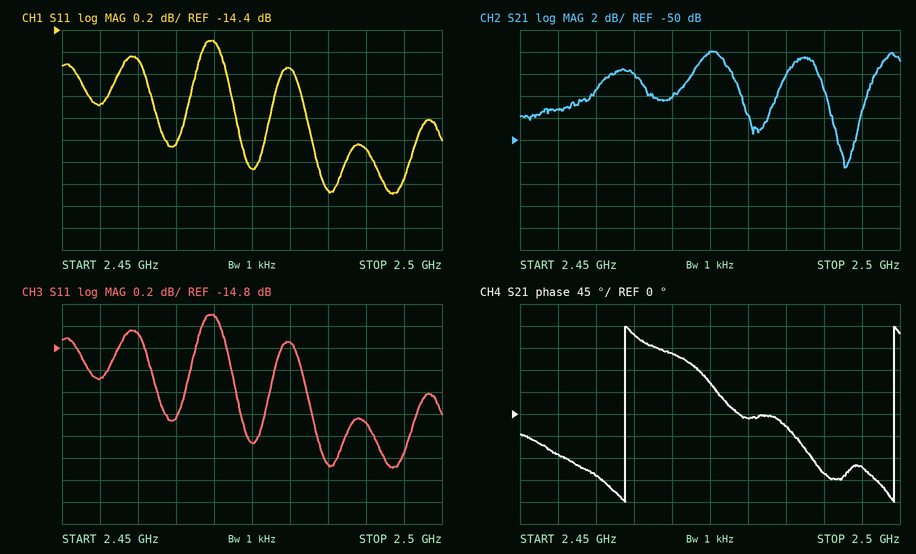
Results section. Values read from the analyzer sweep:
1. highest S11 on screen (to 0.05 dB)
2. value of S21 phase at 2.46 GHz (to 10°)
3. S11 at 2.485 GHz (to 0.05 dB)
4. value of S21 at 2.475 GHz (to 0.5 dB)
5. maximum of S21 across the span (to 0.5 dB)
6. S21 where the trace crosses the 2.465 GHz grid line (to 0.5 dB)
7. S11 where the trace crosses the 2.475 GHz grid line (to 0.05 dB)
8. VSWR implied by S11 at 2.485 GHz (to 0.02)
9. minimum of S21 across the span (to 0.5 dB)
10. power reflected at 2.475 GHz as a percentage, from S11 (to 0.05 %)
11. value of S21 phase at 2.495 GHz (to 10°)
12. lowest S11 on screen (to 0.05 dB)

-14.50 dB
-130°
-15.85 dB
-42.0 dB
-42.0 dB
-44.0 dB
-15.65 dB
1.38
-52.5 dB
2.70 %
-110°
-15.90 dB
